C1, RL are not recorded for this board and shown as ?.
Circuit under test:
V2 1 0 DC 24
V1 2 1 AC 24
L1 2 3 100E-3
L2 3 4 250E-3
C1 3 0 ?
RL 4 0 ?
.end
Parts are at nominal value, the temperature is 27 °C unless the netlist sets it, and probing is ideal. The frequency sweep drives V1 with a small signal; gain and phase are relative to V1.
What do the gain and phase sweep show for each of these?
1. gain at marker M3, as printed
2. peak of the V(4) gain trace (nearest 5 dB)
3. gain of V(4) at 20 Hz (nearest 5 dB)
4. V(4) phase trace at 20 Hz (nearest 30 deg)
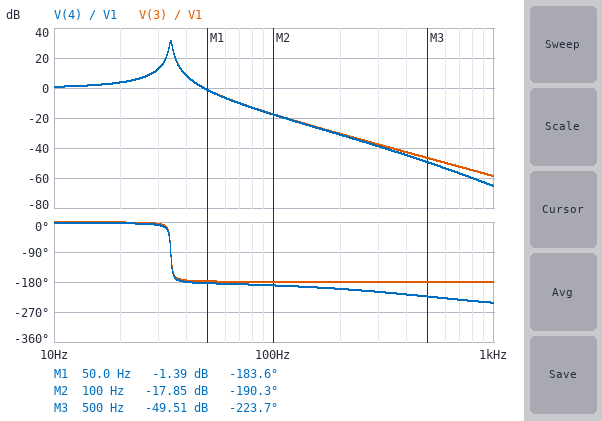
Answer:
-49.51 dB
30 dB
5 dB
0 deg
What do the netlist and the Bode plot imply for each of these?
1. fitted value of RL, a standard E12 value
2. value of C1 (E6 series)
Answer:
820 Ω
220 µF
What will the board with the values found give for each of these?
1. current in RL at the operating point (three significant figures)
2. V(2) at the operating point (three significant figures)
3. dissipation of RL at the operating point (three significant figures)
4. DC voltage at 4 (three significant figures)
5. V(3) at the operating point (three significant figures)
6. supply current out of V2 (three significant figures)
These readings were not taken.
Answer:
29.3 mA
24.0 V
702 mW
24.0 V
24.0 V
29.3 mA
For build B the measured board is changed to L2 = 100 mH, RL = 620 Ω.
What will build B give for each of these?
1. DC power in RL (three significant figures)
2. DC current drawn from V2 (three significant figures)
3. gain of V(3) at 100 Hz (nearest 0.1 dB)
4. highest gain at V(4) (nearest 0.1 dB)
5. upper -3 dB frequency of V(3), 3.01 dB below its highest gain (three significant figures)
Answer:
929 mW
38.7 mA
-17.7 dB
29.3 dB
34.5 Hz
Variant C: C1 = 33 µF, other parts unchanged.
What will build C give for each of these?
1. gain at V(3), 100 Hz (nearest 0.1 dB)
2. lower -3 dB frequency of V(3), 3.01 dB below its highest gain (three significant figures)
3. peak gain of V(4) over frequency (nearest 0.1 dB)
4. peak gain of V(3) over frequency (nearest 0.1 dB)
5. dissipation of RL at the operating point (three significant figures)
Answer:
10.5 dB
85.1 Hz
23.5 dB
23.7 dB
702 mW
